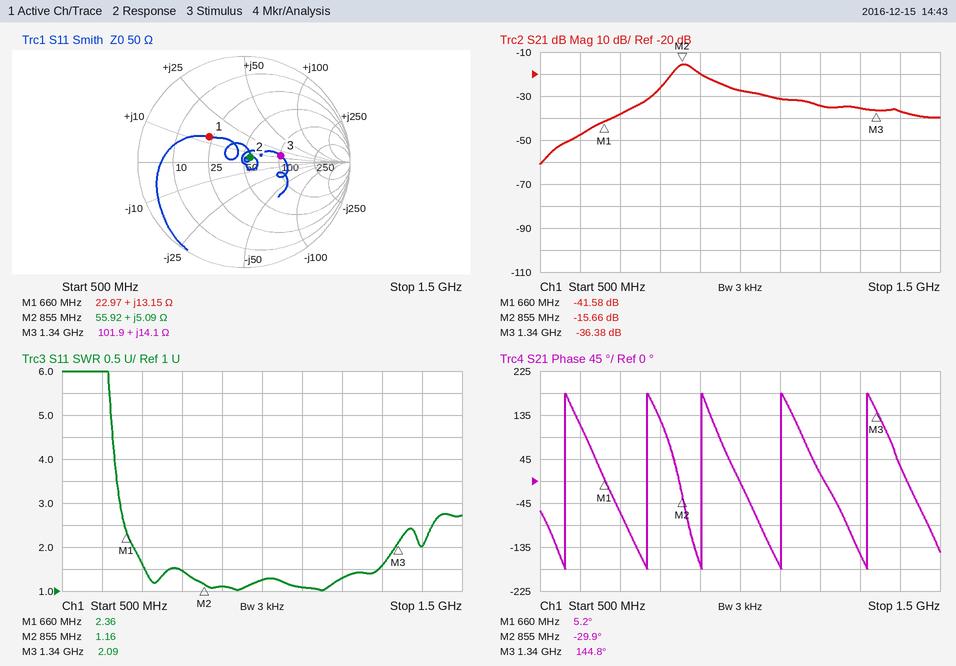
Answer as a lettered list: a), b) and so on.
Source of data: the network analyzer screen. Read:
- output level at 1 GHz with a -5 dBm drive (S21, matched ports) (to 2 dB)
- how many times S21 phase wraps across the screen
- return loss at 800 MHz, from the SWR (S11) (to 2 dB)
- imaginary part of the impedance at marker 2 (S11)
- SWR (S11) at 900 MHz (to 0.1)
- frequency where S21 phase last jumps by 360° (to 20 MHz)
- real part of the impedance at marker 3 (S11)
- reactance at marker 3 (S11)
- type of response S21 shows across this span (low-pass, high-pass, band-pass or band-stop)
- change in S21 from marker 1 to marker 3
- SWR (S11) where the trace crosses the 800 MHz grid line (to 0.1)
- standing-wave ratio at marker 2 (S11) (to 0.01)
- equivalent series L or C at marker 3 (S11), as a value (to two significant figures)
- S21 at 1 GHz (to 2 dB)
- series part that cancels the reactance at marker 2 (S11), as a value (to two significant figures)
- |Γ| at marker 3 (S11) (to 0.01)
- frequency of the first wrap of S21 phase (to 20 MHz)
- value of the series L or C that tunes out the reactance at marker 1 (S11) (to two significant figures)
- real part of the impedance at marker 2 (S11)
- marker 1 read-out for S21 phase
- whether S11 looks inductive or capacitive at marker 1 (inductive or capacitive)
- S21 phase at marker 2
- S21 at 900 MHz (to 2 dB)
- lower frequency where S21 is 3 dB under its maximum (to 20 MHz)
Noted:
a) -32 dBm
b) 5
c) 14 dB
d) +5.09 Ω
e) 1.1
f) 1.32 GHz
g) 101.9 Ω
h) +14.1 Ω
i) band-pass
j) 5.20 dB
k) 1.5
l) 1.16
m) 1.7 nH
n) -28 dB
o) 37 pF
p) 0.35
q) 560 MHz
r) 18 pF
s) 55.92 Ω
t) 5.2°
u) inductive
v) -29.9°
w) -20 dB
x) 840 MHz
